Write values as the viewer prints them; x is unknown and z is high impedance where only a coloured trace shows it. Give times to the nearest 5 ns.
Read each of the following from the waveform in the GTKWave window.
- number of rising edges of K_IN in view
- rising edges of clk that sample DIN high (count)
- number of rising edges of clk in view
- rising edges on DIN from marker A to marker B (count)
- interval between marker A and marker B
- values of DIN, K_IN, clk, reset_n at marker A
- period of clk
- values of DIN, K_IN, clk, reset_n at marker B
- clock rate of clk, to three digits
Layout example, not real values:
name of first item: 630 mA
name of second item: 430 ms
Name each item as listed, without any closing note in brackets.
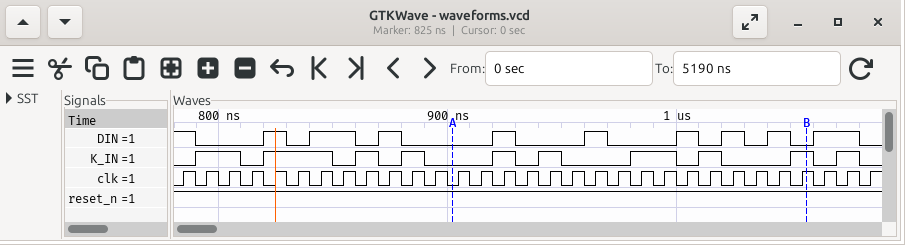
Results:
number of rising edges of K_IN in view: 10
rising edges of clk that sample DIN high: 12
number of rising edges of clk in view: 31
rising edges on DIN from marker A to marker B: 5
interval between marker A and marker B: 155 ns
values of DIN, K_IN, clk, reset_n at marker A: DIN=0, K_IN=0, clk=0, reset_n=1
period of clk: 10 ns
values of DIN, K_IN, clk, reset_n at marker B: DIN=0, K_IN=1, clk=1, reset_n=1
clock rate of clk, to three digits: 100 MHz
